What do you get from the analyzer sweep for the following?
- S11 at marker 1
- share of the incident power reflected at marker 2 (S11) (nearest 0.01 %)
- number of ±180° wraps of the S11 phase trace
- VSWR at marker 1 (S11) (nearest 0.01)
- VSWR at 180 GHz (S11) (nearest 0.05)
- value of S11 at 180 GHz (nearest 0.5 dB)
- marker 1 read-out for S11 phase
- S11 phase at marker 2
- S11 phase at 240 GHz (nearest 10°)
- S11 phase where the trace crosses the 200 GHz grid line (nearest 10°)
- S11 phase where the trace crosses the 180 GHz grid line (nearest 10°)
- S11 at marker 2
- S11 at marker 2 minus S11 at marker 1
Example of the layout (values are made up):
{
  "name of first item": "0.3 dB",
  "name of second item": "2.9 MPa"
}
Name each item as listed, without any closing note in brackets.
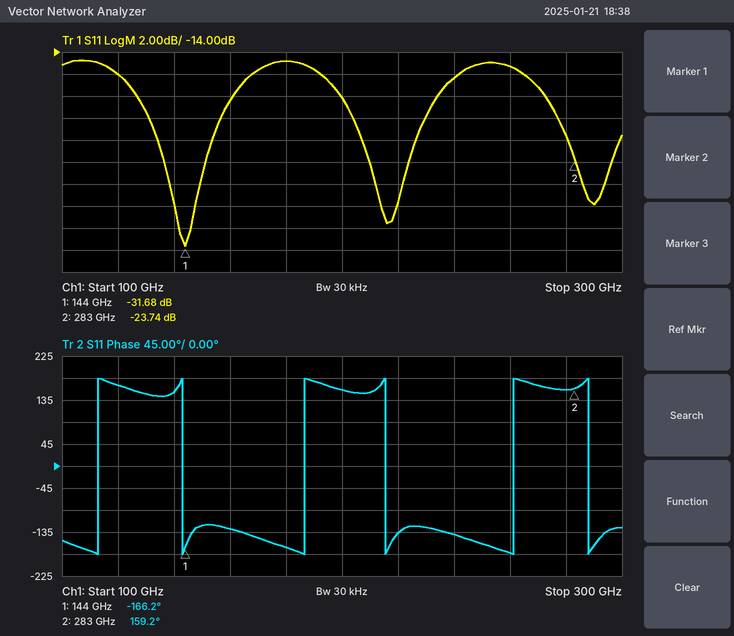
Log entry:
{
  "S11 at marker 1": "-31.68 dB",
  "share of the incident power reflected at marker 2 (S11)": "0.42 %",
  "number of ±180° wraps of the S11 phase trace": "6",
  "VSWR at marker 1 (S11)": "1.05",
  "VSWR at 180 GHz (S11)": "1.45",
  "value of S11 at 180 GHz": "-15.0 dB",
  "marker 1 read-out for S11 phase": "-166.2°",
  "S11 phase at marker 2": "159.2°",
  "S11 phase at 240 GHz": "-140°",
  "S11 phase where the trace crosses the 200 GHz grid line": "160°",
  "S11 phase where the trace crosses the 180 GHz grid line": "-170°",
  "S11 at marker 2": "-23.74 dB",
  "S11 at marker 2 minus S11 at marker 1": "7.94 dB"
}
